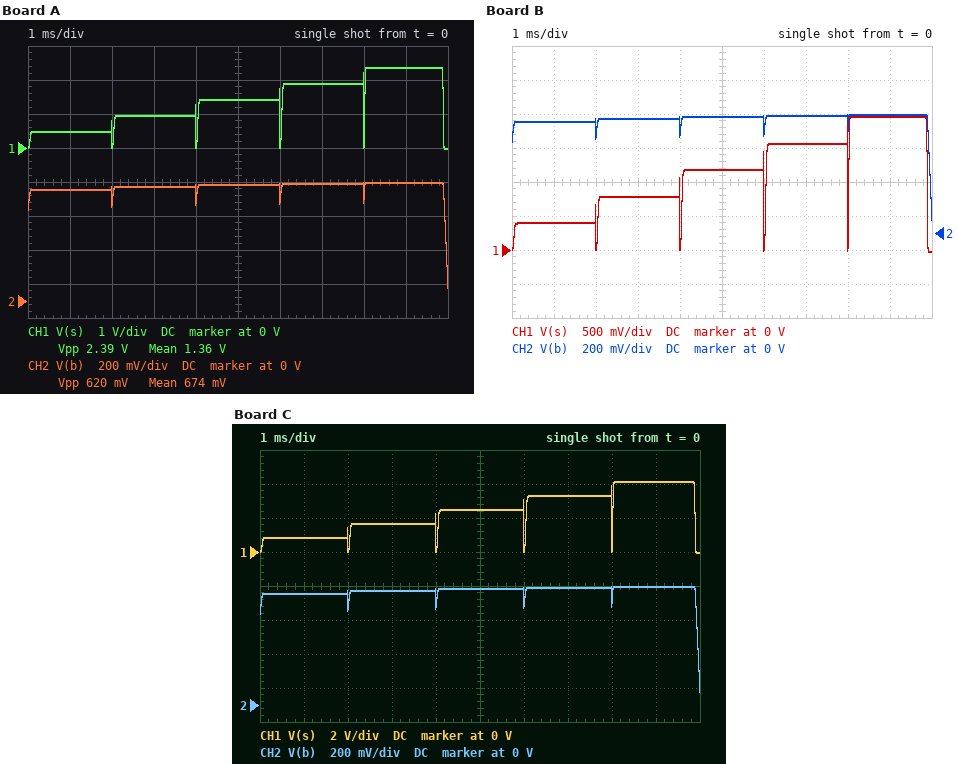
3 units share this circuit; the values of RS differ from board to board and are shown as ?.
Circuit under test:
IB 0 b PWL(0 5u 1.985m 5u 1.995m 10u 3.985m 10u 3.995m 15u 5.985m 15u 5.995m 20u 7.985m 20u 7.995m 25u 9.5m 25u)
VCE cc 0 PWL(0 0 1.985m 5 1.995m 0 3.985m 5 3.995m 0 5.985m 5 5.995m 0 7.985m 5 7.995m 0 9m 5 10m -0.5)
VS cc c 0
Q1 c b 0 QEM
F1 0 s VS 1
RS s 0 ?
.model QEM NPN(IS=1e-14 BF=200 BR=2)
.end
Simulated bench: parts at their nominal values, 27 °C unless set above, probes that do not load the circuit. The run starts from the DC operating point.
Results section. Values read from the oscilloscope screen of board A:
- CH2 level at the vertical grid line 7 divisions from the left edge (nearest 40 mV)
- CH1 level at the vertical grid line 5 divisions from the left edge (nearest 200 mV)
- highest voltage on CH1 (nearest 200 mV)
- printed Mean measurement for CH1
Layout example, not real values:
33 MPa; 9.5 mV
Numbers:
680 mV; 1.4 V; 2.4 V; 1.36 V
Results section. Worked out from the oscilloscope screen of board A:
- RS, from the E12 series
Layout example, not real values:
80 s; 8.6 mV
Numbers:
470 Ω
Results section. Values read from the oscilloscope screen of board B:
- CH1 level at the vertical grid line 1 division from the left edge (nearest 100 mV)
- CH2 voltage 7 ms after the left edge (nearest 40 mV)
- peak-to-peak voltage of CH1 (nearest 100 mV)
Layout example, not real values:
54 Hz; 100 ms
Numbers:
400 mV; 680 mV; 2.0 V
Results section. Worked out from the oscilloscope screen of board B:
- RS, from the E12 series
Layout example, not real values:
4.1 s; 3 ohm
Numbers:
390 Ω
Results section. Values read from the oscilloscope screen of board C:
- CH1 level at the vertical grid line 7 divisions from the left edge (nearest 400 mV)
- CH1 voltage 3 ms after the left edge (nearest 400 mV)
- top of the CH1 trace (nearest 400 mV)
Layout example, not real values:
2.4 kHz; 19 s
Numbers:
3.2 V; 1.6 V; 4.0 V
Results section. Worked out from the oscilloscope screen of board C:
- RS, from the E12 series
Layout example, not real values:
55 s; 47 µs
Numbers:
820 Ω
